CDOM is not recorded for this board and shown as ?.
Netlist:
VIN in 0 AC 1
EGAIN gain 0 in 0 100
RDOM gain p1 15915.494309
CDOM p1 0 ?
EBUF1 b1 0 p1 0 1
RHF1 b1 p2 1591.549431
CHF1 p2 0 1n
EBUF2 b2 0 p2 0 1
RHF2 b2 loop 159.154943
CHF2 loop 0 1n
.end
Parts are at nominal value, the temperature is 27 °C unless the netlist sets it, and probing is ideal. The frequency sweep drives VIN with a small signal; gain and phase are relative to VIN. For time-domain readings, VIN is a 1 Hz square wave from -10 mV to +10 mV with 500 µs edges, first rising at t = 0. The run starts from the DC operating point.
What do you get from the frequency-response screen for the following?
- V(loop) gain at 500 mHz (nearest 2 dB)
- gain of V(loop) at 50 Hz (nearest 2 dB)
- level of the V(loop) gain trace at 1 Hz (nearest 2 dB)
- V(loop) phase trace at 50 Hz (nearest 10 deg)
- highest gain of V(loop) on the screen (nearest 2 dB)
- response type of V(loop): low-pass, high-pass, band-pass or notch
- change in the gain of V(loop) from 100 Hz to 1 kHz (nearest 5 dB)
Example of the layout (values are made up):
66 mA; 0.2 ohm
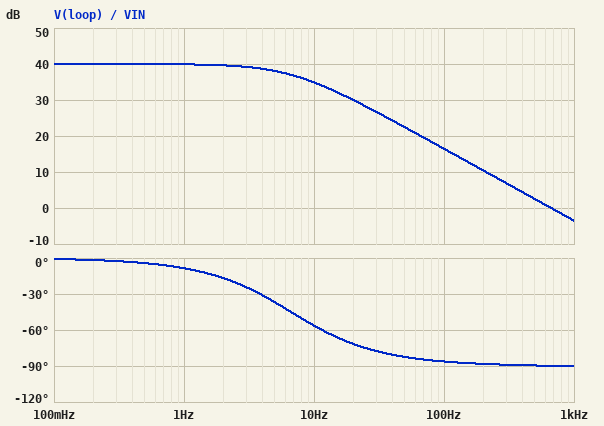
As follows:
40 dB; 22 dB; 40 dB; -80 deg; 40 dB; low-pass; -20 dB
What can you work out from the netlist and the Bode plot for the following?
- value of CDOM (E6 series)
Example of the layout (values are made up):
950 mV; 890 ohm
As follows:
1.5 µF
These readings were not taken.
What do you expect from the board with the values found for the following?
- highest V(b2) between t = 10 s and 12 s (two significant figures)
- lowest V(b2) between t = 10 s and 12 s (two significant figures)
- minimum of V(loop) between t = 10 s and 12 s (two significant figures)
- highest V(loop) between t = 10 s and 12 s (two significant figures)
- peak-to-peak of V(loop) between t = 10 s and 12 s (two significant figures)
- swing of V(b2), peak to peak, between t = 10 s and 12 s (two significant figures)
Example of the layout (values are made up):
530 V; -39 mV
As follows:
1.0 V; -1.0 V; -1.0 V; 1.0 V; 2.0 V; 2.0 V
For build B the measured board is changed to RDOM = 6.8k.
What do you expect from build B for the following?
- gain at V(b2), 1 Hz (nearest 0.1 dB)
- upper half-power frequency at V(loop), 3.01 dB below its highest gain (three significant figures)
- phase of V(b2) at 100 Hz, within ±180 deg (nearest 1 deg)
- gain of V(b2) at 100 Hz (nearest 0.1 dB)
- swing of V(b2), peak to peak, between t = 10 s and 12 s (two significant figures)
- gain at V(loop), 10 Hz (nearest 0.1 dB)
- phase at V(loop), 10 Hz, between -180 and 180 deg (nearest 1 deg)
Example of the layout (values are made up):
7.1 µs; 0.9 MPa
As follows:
40.0 dB; 15.6 Hz; -81 deg; 23.8 dB; 2.0 V; 38.5 dB; -33 deg
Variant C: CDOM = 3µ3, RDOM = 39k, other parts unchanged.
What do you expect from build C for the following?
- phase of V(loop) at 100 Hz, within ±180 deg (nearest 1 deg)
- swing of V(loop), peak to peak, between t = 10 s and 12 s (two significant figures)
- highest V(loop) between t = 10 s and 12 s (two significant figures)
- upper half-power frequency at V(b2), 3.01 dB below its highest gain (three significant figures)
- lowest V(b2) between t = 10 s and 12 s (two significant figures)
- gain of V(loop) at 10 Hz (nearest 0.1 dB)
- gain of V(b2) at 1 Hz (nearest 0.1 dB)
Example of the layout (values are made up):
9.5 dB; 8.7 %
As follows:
-89 deg; 1.9 V; 960 mV; 1.24 Hz; -960 mV; 21.8 dB; 37.8 dB
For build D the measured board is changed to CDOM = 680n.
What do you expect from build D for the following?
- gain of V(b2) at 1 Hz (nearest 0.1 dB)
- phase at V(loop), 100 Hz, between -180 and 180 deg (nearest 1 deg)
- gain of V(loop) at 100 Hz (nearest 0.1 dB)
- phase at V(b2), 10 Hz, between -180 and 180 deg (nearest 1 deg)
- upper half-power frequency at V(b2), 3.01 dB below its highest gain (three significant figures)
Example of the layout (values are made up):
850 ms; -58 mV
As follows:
40.0 dB; -82 deg; 23.3 dB; -34 deg; 14.7 Hz
